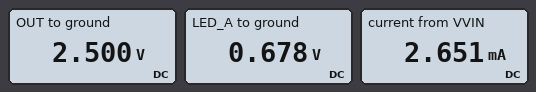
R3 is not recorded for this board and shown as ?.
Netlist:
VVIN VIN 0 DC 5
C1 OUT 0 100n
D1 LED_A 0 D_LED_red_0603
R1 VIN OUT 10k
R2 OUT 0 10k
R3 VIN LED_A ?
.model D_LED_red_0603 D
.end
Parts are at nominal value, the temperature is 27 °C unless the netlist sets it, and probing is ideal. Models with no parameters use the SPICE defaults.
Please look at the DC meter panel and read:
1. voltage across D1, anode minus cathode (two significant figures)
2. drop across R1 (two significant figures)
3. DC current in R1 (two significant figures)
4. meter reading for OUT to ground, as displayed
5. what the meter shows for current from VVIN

680 mV
2.5 V
250 µA
2.500 V
2.651 mA
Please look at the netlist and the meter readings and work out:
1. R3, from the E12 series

1.8 kΩ
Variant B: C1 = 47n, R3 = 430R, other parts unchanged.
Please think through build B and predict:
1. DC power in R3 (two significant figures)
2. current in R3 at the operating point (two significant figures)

43 mW
10 mA
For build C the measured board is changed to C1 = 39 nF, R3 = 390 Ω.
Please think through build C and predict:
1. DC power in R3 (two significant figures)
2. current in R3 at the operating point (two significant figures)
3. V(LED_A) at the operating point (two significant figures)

47 mW
11 mA
720 mV
